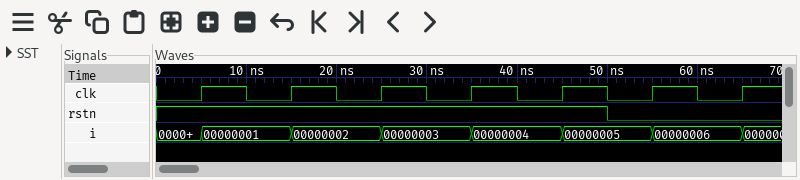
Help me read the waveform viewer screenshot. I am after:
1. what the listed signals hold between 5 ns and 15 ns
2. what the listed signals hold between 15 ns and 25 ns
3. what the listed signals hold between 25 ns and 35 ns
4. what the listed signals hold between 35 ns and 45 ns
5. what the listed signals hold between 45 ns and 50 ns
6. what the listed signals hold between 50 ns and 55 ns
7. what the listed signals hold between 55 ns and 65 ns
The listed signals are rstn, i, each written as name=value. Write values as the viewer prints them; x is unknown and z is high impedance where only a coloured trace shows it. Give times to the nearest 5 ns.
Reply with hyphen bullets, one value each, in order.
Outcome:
- rstn=1, i=00000001
- rstn=1, i=00000002
- rstn=1, i=00000003
- rstn=1, i=00000004
- rstn=1, i=00000005
- rstn=0, i=00000005
- rstn=0, i=00000006
